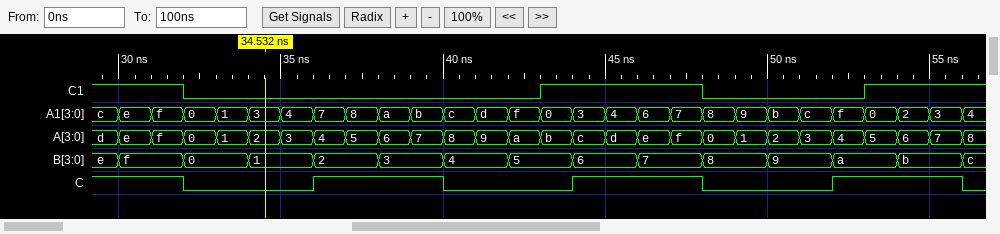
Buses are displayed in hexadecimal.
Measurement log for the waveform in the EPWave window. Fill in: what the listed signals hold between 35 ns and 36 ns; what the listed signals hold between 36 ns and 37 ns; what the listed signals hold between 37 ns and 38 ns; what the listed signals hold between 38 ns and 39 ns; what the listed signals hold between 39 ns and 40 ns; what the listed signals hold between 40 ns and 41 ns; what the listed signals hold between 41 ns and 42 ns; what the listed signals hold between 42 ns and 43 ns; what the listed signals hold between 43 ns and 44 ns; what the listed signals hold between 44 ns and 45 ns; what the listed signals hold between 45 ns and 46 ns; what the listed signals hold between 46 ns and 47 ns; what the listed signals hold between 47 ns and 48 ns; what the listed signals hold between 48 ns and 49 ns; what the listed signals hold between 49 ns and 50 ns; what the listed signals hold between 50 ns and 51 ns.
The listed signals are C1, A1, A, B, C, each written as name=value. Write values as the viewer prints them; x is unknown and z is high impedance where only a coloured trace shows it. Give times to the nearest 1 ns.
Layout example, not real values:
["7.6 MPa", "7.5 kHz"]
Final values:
["C1=0, A1=4, A=3, B=1, C=0", "C1=0, A1=7, A=4, B=2, C=1", "C1=0, A1=8, A=5, B=2, C=1", "C1=0, A1=a, A=6, B=3, C=1", "C1=0, A1=b, A=7, B=3, C=1", "C1=0, A1=c, A=8, B=4, C=0", "C1=0, A1=d, A=9, B=4, C=0", "C1=0, A1=f, A=a, B=5, C=0", "C1=1, A1=0, A=b, B=5, C=0", "C1=1, A1=3, A=c, B=6, C=1", "C1=1, A1=4, A=d, B=6, C=1", "C1=1, A1=6, A=e, B=7, C=1", "C1=1, A1=7, A=f, B=7, C=1", "C1=0, A1=8, A=0, B=8, C=0", "C1=0, A1=9, A=1, B=8, C=0", "C1=0, A1=b, A=2, B=9, C=0"]
